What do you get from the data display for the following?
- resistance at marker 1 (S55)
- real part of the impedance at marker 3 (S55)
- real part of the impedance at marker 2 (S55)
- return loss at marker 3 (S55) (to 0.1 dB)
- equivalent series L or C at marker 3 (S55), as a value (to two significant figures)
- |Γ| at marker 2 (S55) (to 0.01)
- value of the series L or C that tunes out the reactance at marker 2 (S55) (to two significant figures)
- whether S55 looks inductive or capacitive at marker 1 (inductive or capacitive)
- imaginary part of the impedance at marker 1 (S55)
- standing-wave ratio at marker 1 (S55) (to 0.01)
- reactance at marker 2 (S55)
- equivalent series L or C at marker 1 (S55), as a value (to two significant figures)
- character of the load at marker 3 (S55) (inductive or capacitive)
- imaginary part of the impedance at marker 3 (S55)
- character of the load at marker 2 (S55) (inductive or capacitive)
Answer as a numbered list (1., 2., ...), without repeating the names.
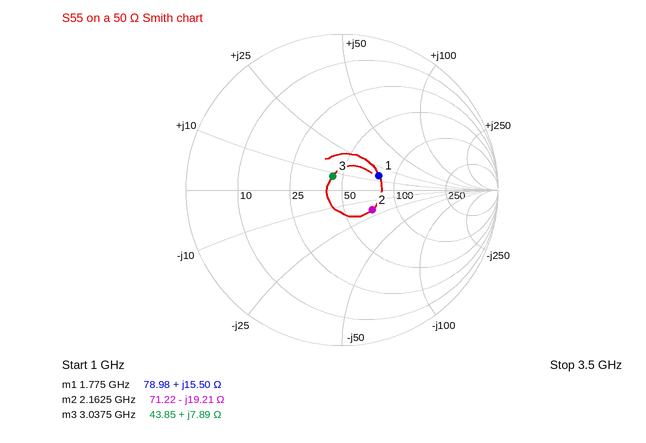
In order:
1. 78.98 Ω
2. 43.85 Ω
3. 71.22 Ω
4. 19.5 dB
5. 410 pH
6. 0.23
7. 1.4 nH
8. inductive
9. +15.50 Ω
10. 1.68
11. -19.21 Ω
12. 1.4 nH
13. inductive
14. +7.89 Ω
15. capacitive
